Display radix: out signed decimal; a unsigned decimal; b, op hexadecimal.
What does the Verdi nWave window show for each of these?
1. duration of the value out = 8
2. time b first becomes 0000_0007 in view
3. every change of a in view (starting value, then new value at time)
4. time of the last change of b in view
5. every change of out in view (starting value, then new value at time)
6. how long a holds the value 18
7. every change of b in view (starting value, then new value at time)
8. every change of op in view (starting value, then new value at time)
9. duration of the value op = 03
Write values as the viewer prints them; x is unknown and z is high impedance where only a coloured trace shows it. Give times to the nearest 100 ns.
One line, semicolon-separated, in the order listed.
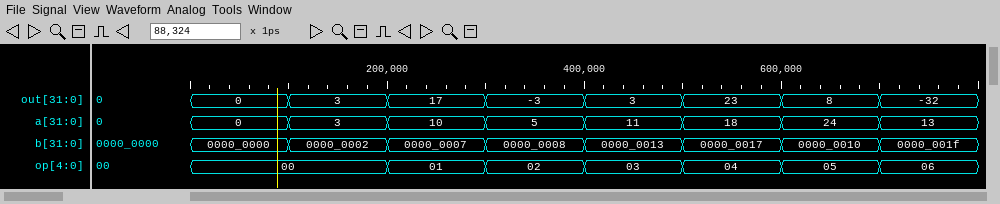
100 ns; 200 ns; 0, 3 at 100 ns, 10 at 200 ns, 5 at 300 ns, 11 at 400 ns, 18 at 500 ns, 24 at 600 ns, 13 at 700 ns; 700 ns; 0, 3 at 100 ns, 17 at 200 ns, -3 at 300 ns, 3 at 400 ns, 23 at 500 ns, 8 at 600 ns, -32 at 700 ns; 100 ns; 0000_0000, 0000_0002 at 100 ns, 0000_0007 at 200 ns, 0000_0008 at 300 ns, 0000_0013 at 400 ns, 0000_0017 at 500 ns, 0000_0010 at 600 ns, 0000_001f at 700 ns; 00, 01 at 200 ns, 02 at 300 ns, 03 at 400 ns, 04 at 500 ns, 05 at 600 ns, 06 at 700 ns; 100 ns
